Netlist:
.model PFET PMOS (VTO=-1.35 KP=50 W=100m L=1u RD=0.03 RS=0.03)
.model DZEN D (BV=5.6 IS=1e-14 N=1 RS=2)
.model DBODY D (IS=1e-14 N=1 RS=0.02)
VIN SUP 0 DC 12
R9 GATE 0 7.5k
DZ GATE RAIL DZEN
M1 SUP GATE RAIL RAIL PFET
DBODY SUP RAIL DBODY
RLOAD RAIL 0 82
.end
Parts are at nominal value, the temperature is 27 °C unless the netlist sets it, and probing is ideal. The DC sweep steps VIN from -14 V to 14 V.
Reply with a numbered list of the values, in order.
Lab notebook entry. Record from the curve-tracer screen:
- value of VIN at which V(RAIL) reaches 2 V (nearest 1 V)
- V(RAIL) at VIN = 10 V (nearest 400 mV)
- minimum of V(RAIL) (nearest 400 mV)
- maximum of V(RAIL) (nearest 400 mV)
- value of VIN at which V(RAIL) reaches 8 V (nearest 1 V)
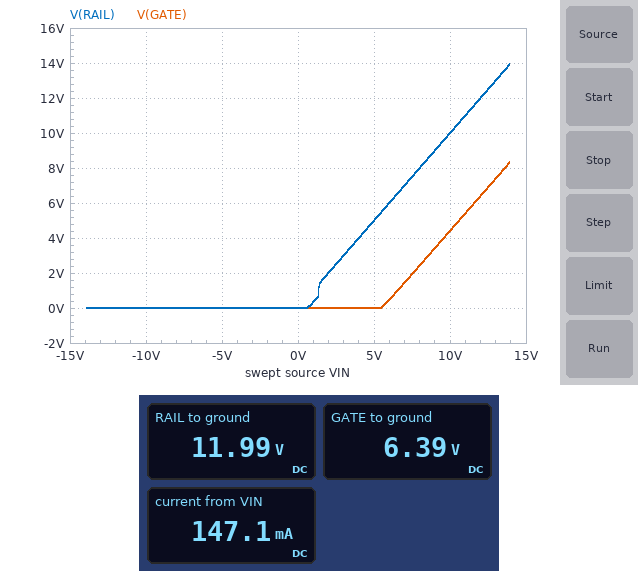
1. 2 V
2. 10.0 V
3. 0 V
4. 14.0 V
5. 8 V
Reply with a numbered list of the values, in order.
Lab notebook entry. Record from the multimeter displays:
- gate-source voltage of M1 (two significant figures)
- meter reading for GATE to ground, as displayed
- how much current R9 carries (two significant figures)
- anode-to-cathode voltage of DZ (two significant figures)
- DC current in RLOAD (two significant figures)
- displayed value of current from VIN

1. -5.6 V
2. 6.39 V
3. 850 µA
4. -5.6 V
5. 150 mA
6. 147.1 mA
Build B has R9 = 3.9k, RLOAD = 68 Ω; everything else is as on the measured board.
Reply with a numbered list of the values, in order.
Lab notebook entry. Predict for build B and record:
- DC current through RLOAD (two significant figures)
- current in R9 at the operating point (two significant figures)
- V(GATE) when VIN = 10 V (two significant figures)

1. 180 mA
2. 1.6 mA
3. 4.4 V
